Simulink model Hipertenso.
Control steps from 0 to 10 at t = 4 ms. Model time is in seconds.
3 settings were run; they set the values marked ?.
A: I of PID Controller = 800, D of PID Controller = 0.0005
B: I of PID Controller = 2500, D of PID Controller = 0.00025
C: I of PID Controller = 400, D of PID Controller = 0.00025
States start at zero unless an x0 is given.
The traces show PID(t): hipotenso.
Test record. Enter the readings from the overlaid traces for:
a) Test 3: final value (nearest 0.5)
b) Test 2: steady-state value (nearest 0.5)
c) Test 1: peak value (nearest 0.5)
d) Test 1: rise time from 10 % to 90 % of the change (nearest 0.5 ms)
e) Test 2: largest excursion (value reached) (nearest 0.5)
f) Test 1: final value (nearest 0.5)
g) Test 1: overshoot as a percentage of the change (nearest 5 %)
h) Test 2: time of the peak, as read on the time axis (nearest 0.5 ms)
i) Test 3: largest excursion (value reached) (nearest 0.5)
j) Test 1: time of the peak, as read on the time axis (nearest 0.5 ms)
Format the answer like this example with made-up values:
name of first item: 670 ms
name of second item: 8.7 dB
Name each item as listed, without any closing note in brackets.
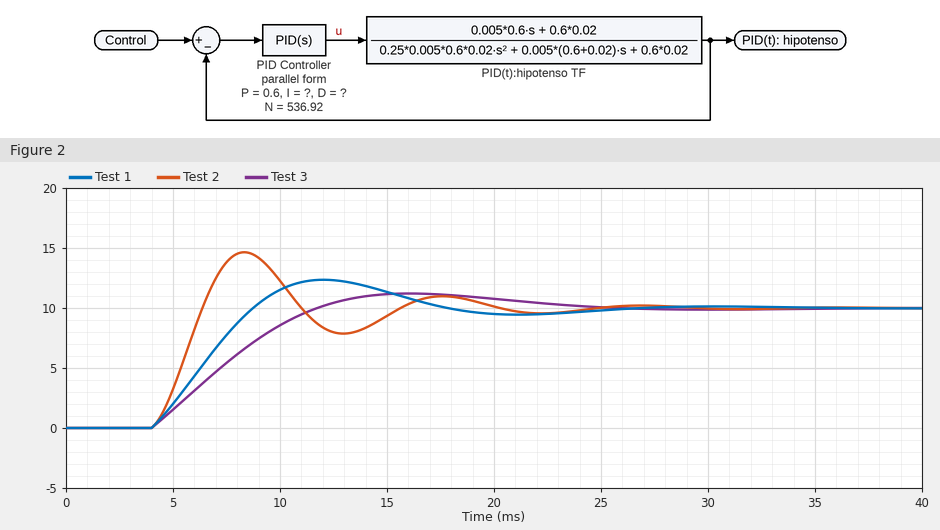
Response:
Test 3: final value: 10.0
Test 2: steady-state value: 10.0
Test 1: peak value: 12.5
Test 1: rise time from 10 % to 90 % of the change: 3.5 ms
Test 2: largest excursion (value reached): 14.5
Test 1: final value: 10.0
Test 1: overshoot as a percentage of the change: 25 %
Test 2: time of the peak, as read on the time axis: 8.5 ms
Test 3: largest excursion (value reached): 11.0
Test 1: time of the peak, as read on the time axis: 12.0 ms
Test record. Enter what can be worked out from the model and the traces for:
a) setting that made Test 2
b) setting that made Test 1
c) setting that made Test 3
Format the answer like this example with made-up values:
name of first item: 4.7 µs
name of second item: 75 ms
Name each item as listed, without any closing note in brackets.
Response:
setting that made Test 2: B
setting that made Test 1: A
setting that made Test 3: C
